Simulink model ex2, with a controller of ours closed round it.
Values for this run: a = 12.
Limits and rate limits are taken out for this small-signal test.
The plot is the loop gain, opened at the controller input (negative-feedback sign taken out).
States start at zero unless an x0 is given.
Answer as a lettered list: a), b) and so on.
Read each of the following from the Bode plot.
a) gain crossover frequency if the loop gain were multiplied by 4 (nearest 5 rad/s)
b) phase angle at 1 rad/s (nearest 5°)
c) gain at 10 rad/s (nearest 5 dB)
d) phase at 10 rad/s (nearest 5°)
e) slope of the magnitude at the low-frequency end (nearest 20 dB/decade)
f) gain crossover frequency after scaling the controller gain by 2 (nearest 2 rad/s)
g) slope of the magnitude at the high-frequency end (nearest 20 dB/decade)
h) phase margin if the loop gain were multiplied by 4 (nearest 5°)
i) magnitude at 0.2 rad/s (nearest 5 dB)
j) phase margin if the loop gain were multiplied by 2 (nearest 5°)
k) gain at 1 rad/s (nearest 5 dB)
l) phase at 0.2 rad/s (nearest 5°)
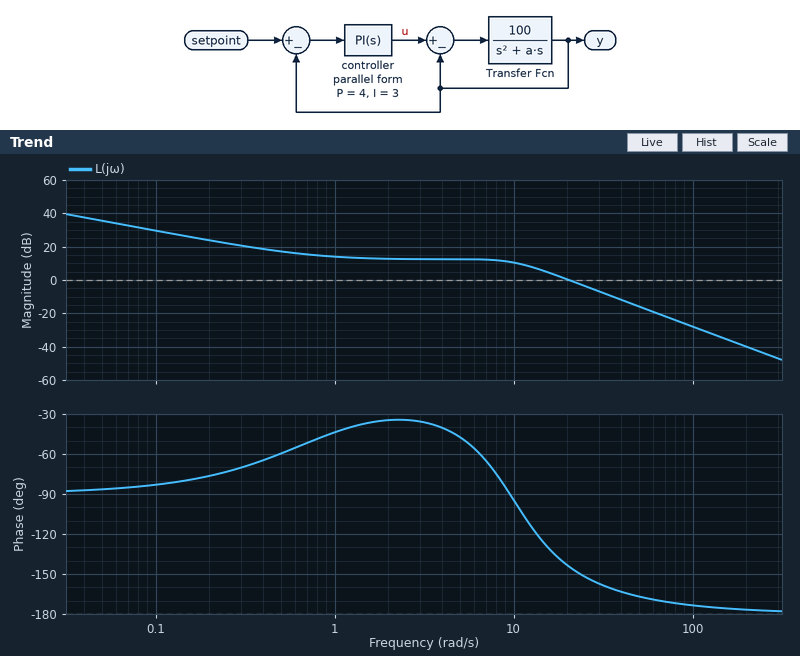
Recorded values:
a) 40 rad/s
b) -45°
c) 10 dB
d) -95°
e) -20 dB/decade
f) 28 rad/s
g) -40 dB/decade
h) 15°
i) 25 dB
j) 25°
k) 15 dB
l) -75°
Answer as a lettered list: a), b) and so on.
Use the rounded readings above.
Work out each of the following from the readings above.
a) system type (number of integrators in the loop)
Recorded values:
a) 1
